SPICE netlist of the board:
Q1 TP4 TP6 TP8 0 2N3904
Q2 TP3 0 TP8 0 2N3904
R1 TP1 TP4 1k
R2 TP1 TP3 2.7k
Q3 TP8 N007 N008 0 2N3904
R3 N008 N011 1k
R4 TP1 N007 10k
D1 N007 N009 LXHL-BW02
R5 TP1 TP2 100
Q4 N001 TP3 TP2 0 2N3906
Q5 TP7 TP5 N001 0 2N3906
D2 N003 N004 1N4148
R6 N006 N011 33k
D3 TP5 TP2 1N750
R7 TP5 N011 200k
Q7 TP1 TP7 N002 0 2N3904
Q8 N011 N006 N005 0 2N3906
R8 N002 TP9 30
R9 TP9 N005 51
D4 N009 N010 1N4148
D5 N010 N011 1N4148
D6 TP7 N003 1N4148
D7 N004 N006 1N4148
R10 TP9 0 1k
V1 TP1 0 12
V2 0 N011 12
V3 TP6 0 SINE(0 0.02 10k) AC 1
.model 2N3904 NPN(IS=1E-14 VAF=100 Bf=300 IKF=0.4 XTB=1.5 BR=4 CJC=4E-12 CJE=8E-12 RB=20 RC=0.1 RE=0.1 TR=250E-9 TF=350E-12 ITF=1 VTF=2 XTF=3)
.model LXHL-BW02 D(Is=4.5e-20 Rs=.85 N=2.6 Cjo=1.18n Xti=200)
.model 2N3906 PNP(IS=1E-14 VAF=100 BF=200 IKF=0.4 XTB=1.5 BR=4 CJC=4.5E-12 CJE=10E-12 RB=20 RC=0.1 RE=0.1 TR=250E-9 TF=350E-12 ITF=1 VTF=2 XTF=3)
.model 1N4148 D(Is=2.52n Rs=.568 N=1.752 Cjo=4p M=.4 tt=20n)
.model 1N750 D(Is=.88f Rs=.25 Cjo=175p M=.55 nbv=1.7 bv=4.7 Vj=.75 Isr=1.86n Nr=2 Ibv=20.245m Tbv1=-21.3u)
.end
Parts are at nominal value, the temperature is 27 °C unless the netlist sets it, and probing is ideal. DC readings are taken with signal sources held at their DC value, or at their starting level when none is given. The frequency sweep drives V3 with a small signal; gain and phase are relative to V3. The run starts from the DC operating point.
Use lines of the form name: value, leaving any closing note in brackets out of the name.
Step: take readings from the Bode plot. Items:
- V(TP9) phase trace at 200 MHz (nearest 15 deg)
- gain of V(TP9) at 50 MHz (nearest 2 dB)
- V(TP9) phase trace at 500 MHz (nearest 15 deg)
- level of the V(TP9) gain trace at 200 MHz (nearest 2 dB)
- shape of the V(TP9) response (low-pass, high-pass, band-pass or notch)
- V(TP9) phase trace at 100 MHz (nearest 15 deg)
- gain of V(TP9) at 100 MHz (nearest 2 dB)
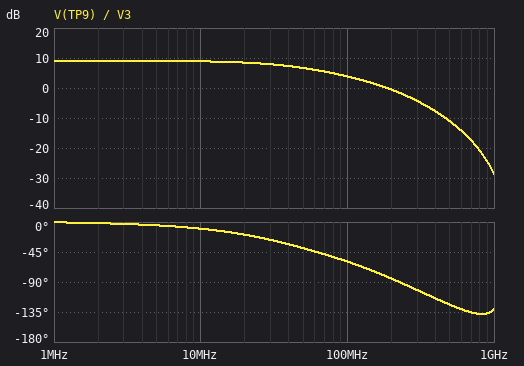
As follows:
V(TP9) phase trace at 200 MHz: -90 deg
gain of V(TP9) at 50 MHz: 6 dB
V(TP9) phase trace at 500 MHz: -120 deg
level of the V(TP9) gain trace at 200 MHz: 0 dB
shape of the V(TP9) response: low-pass
V(TP9) phase trace at 100 MHz: -60 deg
gain of V(TP9) at 100 MHz: 4 dB
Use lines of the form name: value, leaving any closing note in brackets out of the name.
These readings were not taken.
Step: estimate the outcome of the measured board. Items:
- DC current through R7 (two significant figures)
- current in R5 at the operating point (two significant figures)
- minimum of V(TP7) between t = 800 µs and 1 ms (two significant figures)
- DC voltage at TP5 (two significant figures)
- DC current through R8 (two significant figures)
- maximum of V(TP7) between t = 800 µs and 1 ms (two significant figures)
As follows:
DC current through R7: 120 µA
current in R5 at the operating point: 2.0 mA
minimum of V(TP7) between t = 800 µs and 1 ms: 12 V
DC voltage at TP5: 11 V
DC current through R8: 11 mA
maximum of V(TP7) between t = 800 µs and 1 ms: 12 V
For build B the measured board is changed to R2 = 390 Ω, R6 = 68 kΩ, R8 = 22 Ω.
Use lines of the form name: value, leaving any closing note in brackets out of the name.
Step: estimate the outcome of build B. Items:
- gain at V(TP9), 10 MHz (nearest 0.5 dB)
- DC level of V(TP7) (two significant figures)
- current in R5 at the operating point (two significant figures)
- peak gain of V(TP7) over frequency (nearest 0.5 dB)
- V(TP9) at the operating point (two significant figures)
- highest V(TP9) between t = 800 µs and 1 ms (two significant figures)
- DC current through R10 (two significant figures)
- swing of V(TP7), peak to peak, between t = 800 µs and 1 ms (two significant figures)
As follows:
gain at V(TP9), 10 MHz: 33.0 dB
DC level of V(TP7): -3.5 V
current in R5 at the operating point: 180 µA
peak gain of V(TP7) over frequency: 63.5 dB
V(TP9) at the operating point: -4.0 V
highest V(TP9) between t = 800 µs and 1 ms: 11 V
DC current through R10: 4.0 mA
swing of V(TP7), peak to peak, between t = 800 µs and 1 ms: 21 V
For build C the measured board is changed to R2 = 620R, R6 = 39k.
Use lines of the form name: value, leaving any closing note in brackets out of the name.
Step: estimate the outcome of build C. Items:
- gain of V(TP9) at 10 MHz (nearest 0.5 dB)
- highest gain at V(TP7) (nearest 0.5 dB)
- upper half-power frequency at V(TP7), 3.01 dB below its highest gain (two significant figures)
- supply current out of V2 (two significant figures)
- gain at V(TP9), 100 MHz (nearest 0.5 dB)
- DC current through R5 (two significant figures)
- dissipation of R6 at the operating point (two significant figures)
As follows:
gain of V(TP9) at 10 MHz: 8.0 dB
highest gain at V(TP7): 8.5 dB
upper half-power frequency at V(TP7), 3.01 dB below its highest gain: 55 MHz
supply current out of V2: 6.1 mA
gain at V(TP9), 100 MHz: 3.0 dB
DC current through R5: 1.0 mA
dissipation of R6 at the operating point: 13 mW
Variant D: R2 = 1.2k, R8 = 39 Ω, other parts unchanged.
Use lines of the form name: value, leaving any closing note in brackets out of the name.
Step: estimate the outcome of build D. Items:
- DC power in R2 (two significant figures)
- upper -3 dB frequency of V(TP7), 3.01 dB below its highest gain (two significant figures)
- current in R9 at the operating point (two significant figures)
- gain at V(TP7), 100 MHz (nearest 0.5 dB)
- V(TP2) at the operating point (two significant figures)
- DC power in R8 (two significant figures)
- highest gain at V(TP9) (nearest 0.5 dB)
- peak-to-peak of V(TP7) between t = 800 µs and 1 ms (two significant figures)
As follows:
DC power in R2: 640 µW
upper -3 dB frequency of V(TP7), 3.01 dB below its highest gain: 59 MHz
current in R9 at the operating point: 33 µA
gain at V(TP7), 100 MHz: 3.5 dB
V(TP2) at the operating point: 12 V
DC power in R8: 4.5 mW
highest gain at V(TP9): 8.5 dB
peak-to-peak of V(TP7) between t = 800 µs and 1 ms: 92 mV
